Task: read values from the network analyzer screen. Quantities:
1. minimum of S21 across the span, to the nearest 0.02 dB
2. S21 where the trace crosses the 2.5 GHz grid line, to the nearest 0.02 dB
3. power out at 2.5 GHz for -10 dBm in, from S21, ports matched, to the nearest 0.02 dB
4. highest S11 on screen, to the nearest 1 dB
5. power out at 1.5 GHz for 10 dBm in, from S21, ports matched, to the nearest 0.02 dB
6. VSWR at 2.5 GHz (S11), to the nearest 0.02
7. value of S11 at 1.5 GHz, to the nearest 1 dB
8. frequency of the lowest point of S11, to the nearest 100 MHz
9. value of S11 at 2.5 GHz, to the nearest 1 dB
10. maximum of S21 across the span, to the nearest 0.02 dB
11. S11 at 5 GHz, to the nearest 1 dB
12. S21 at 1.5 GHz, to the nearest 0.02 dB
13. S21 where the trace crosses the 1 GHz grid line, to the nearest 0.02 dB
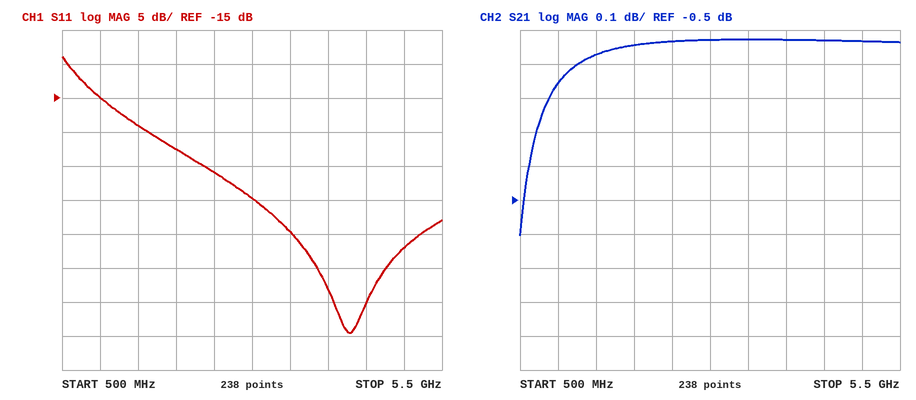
-0.60 dB
-0.04 dB
-10.04 dBm
-9 dB
9.92 dBm
1.10
-19 dB
4.3 GHz
-26 dB
-0.02 dB
-37 dB
-0.08 dB
-0.16 dB
